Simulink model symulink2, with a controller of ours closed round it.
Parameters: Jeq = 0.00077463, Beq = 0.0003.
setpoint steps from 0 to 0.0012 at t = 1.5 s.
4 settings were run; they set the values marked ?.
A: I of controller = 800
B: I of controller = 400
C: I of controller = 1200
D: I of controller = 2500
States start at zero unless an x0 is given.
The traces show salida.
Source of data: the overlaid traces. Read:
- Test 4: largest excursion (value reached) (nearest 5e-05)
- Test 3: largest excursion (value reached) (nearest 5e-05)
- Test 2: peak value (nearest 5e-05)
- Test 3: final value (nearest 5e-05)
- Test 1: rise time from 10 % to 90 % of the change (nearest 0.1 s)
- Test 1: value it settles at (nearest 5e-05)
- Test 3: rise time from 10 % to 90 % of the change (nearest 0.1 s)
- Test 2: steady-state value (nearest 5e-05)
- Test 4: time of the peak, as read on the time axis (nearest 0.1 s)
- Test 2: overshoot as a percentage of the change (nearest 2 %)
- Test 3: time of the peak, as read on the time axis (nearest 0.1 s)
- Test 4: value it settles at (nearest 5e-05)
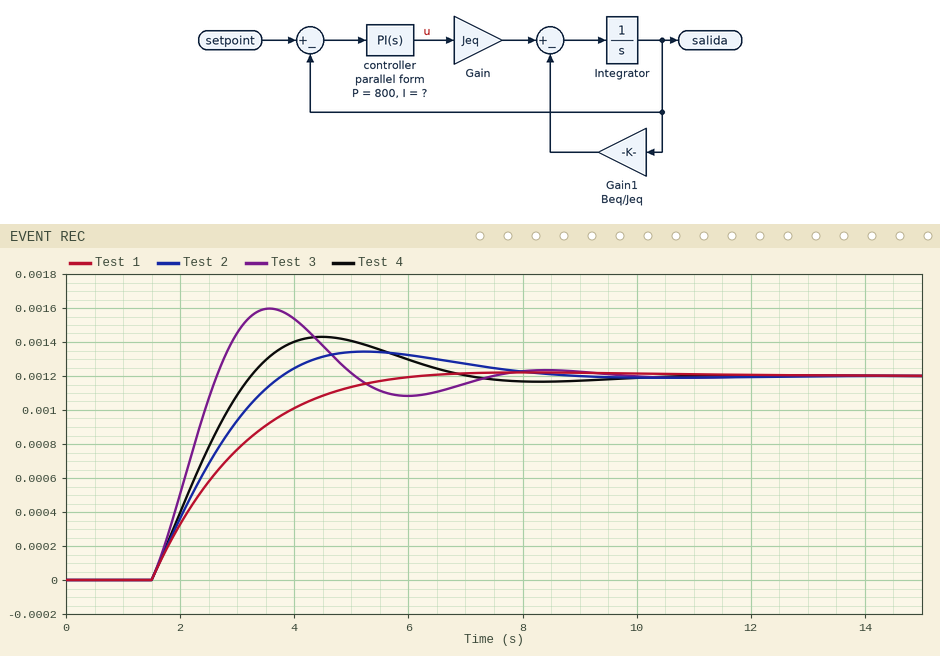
0.00145
0.00160
0.00135
0.00120
2.8 s
0.00120
0.9 s
0.00120
4.5 s
12 %
3.6 s
0.00120
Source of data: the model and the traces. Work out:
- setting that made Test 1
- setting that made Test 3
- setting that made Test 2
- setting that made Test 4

B
D
A
C
